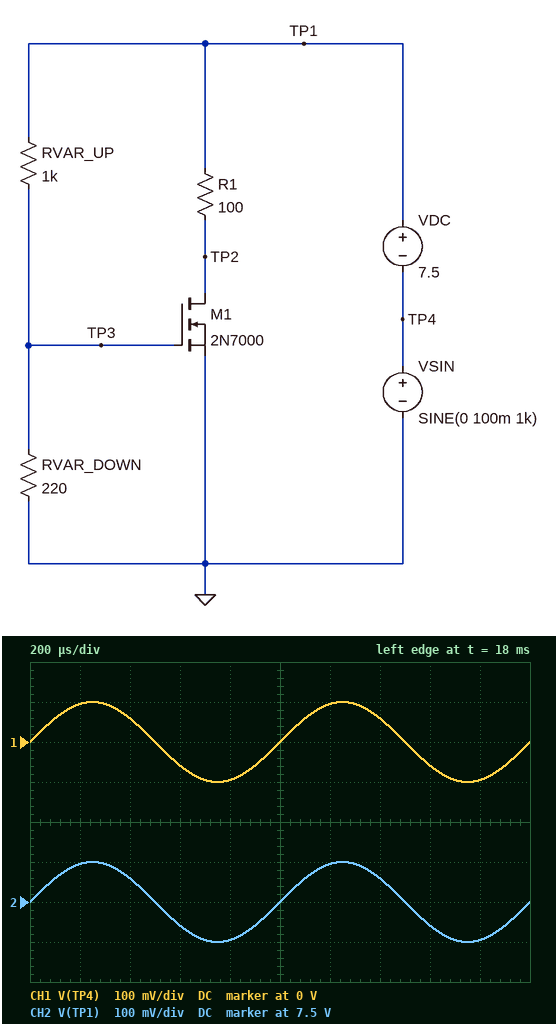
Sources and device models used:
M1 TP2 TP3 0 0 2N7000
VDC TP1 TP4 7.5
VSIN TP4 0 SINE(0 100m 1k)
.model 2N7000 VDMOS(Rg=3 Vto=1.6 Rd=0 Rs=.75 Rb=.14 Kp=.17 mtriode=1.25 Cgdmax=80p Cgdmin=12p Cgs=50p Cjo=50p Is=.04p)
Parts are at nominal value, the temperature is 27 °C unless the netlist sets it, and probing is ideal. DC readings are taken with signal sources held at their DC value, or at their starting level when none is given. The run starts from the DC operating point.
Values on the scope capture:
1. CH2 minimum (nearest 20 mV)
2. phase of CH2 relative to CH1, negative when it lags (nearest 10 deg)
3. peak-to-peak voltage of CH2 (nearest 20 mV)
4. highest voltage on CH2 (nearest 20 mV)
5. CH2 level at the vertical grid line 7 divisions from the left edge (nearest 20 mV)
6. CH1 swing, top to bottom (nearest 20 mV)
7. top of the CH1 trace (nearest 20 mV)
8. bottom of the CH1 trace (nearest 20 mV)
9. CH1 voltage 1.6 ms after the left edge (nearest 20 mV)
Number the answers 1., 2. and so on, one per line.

1. 7.40 V
2. 0 deg
3. 200 mV
4. 7.60 V
5. 7.56 V
6. 200 mV
7. 100 mV
8. -100 mV
9. -60 mV
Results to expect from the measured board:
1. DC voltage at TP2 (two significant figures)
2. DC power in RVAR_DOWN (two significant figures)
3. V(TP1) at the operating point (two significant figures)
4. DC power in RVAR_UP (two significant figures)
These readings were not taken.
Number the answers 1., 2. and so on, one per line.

1. 7.5 V
2. 8.3 mW
3. 7.5 V
4. 38 mW
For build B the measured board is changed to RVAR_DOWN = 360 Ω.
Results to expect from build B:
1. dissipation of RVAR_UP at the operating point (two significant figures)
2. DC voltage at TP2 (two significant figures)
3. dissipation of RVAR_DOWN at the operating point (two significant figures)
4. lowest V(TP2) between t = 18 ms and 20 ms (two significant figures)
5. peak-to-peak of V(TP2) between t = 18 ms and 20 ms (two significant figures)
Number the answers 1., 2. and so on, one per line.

1. 30 mW
2. 6.3 V
3. 11 mW
4. 6.2 V
5. 120 mV
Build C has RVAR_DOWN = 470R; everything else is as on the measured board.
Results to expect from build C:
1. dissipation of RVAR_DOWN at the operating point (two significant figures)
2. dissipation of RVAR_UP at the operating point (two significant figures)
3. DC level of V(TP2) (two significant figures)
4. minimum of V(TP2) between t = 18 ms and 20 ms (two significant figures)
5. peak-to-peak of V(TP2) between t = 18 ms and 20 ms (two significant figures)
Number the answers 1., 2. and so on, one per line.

1. 12 mW
2. 26 mW
3. 2.6 V
4. 2.3 V
5. 550 mV
